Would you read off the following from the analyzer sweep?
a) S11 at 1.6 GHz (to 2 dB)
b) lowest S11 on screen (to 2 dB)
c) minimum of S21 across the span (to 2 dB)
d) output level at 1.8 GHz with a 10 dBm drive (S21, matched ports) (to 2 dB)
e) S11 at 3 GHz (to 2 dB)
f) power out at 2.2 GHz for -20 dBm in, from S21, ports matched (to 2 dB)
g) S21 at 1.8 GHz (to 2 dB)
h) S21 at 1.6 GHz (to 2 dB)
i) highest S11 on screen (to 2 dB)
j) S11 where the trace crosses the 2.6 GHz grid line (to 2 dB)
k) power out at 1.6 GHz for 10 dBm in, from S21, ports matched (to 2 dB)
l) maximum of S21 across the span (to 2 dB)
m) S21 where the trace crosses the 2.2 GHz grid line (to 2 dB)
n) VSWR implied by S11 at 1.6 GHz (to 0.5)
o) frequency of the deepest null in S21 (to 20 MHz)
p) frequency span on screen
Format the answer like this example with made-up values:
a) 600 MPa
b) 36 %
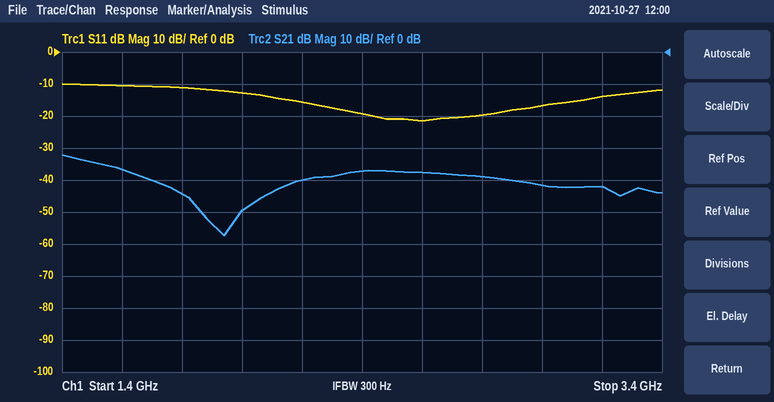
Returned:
a) -10 dB
b) -22 dB
c) -58 dB
d) -34 dBm
e) -16 dB
f) -60 dBm
g) -44 dB
h) -36 dB
i) -10 dB
j) -22 dB
k) -26 dBm
l) -32 dB
m) -40 dB
n) 2.0
o) 1.94 GHz
p) 2 GHz
